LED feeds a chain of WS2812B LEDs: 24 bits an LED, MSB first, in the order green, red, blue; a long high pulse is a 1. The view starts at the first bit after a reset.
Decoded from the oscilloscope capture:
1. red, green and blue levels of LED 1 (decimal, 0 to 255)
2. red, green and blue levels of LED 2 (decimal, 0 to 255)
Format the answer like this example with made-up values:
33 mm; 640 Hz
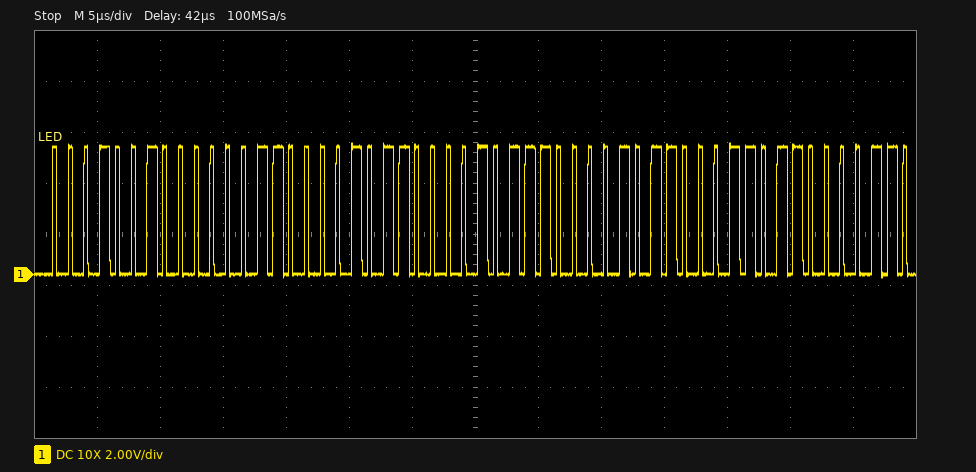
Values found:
6, 18, 22; 11, 23, 27
